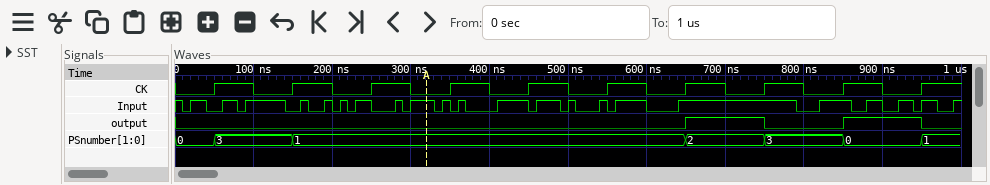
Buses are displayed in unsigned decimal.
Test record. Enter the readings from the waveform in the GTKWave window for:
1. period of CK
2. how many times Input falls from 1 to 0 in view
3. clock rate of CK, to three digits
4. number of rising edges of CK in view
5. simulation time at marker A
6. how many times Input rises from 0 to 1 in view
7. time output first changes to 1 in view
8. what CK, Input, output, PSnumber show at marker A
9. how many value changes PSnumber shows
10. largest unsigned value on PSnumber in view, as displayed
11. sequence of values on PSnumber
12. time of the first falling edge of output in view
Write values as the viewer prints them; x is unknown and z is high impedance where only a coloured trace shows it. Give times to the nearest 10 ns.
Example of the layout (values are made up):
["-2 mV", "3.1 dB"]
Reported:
["100 ns", "22", "10.0 MHz", "10", "320 ns", "22", "650 ns", "CK=0, Input=1, output=0, PSnumber=1", "6", "3", "0, 3, 1, 2, 3, 0, 1", "750 ns"]
